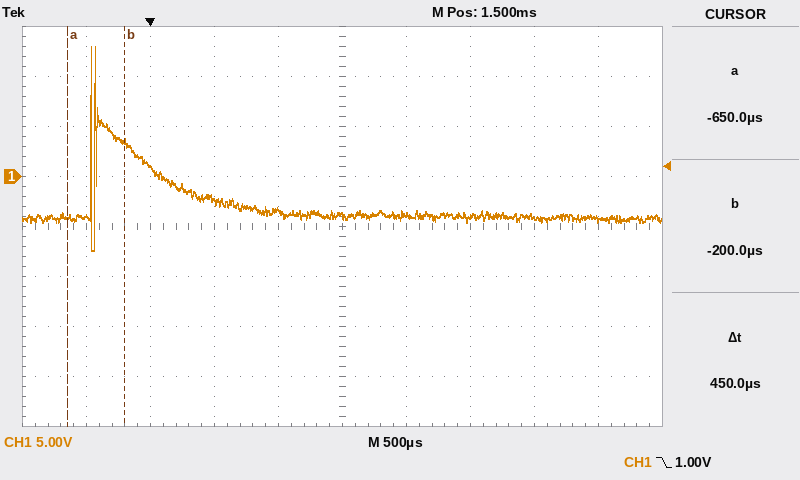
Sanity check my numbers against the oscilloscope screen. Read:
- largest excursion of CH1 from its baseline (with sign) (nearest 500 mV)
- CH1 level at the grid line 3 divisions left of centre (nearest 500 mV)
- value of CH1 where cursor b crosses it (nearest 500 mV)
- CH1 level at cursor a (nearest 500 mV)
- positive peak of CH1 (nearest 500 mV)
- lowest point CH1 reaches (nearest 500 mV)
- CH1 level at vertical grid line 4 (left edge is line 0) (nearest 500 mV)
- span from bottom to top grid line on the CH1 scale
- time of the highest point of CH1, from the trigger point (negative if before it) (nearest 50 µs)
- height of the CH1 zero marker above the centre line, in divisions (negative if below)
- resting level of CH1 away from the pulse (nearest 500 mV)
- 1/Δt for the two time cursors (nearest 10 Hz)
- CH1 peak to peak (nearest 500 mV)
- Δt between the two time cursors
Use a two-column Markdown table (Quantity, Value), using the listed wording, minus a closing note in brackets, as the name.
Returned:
| Quantity | Value |
|---|---|
| largest excursion of CH1 from its baseline (with sign) | +17.0 V |
| CH1 level at the grid line 3 divisions left of centre | 1.0 V |
| value of CH1 where cursor b crosses it | 3.5 V |
| CH1 level at cursor a | -4.0 V |
| positive peak of CH1 | 13.0 V |
| lowest point CH1 reaches | -7.5 V |
| CH1 level at vertical grid line 4 (left edge is line 0) | -3.5 V |
| span from bottom to top grid line on the CH1 scale | 40 V |
| time of the highest point of CH1, from the trigger point (negative if before it) | -450 µs |
| height of the CH1 zero marker above the centre line, in divisions | +1.0 div |
| resting level of CH1 away from the pulse | -4.0 V |
| 1/Δt for the two time cursors | 2.22 kHz |
| CH1 peak to peak | 20.5 V |
| Δt between the two time cursors | 450 µs |
